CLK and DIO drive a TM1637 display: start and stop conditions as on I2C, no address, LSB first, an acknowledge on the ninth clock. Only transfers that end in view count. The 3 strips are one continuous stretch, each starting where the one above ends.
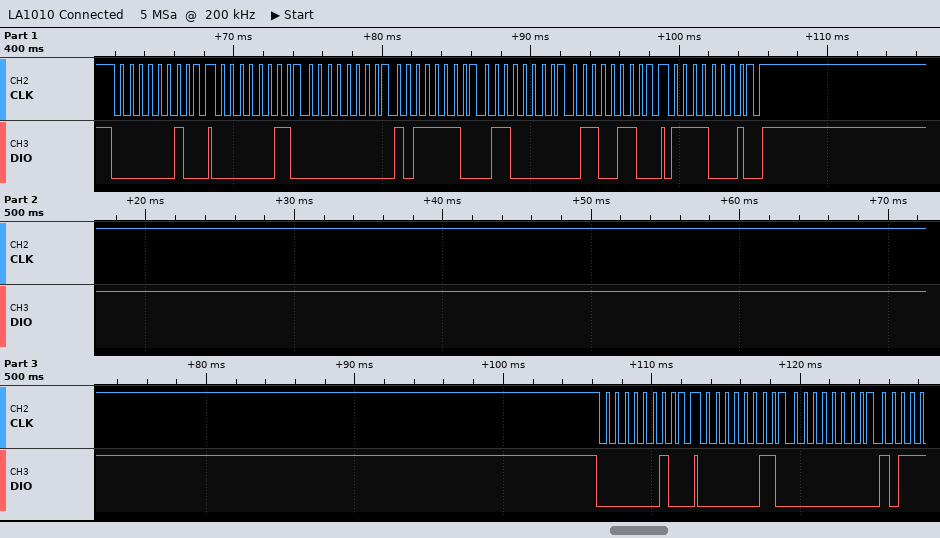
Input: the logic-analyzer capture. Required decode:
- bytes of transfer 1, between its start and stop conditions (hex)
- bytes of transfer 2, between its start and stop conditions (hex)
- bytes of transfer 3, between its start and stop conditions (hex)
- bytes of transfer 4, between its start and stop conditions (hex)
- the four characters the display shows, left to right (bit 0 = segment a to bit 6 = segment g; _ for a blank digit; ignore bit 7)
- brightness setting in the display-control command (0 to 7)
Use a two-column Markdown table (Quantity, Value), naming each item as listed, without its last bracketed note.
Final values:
| Quantity | Value |
|---|---|
| bytes of transfer 1, between its start and stop conditions | 40 |
| bytes of transfer 2, between its start and stop conditions | C0 00 7D 06 66 |
| bytes of transfer 3, between its start and stop conditions | 8F |
| bytes of transfer 4, between its start and stop conditions | 40 |
| the four characters the display shows, left to right | _614 |
| brightness setting in the display-control command | 7 |
